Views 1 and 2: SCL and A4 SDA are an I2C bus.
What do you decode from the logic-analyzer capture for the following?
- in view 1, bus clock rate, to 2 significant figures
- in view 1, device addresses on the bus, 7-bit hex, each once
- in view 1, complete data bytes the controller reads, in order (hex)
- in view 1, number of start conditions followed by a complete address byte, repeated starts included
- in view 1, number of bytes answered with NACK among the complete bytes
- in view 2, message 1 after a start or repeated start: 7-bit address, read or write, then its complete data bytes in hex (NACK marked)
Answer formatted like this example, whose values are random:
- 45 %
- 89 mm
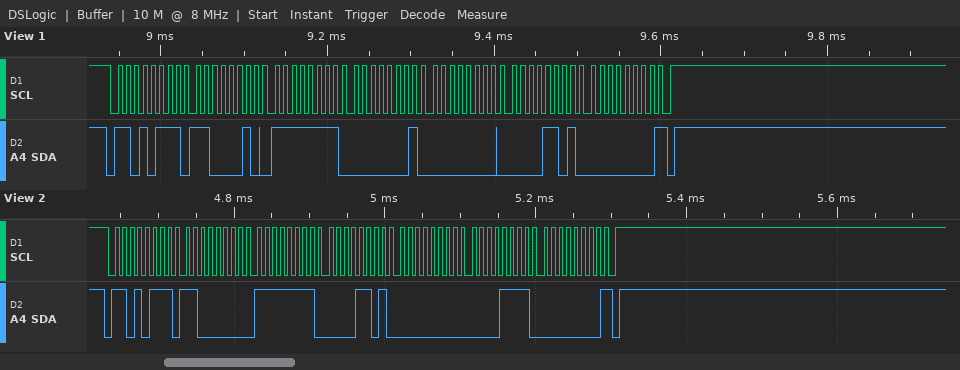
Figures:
- 100 kHz
- 0x6B
- C2 FF 01 00 0D 00
- 1
- 1
- 0x6B read: C0 FF 0D 00 0F 00 NACK
